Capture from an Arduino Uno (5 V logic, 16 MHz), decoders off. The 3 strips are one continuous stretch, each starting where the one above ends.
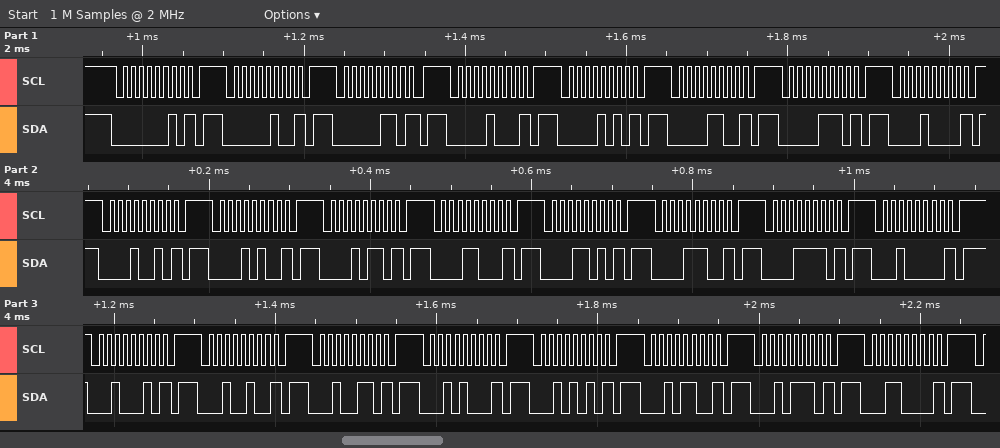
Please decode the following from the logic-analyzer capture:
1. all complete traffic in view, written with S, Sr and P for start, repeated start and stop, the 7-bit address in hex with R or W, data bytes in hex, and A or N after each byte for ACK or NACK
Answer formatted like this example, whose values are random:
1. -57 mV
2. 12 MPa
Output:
1. S 01W N P S 02W N P S 03W N P S 04W N P S 05W N P S 06W N P S 07W N P S 08W N P S 09W N P S 0AW N P S 0BW N P S 0CW N P S 0DW N P S 0EW N P S 0FW N P S 10W N P S 11W N P S 12W N P S 13W N P S 14W N P S 15W N P S 16W N P S 17W N P S 18W N P
